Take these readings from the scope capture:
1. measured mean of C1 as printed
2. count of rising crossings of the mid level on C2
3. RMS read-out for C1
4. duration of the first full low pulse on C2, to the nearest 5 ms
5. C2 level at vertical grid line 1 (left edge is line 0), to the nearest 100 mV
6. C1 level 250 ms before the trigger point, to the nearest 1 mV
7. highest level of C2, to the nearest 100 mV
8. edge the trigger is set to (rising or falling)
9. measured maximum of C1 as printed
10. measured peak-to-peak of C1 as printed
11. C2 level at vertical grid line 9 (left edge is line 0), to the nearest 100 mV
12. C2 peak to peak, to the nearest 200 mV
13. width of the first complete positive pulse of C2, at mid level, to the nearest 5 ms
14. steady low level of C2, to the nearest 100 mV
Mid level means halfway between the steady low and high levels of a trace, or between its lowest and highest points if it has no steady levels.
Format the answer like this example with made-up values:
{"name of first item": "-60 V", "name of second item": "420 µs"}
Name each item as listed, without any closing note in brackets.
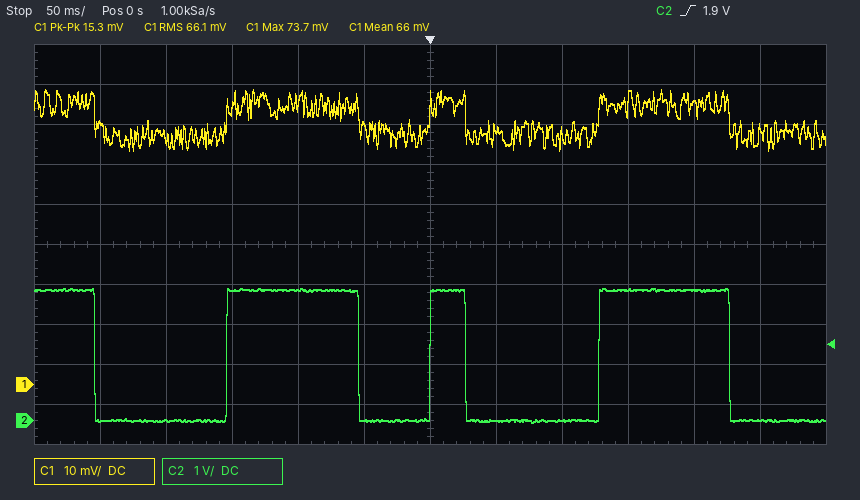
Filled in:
{"measured mean of C1 as printed": "66 mV", "count of rising crossings of the mid level on C2": "3", "RMS read-out for C1": "66.1 mV", "duration of the first full low pulse on C2, to the nearest 5 ms": "100 ms", "C2 level at vertical grid line 1 (left edge is line 0), to the nearest 100 mV": "0.0 V", "C1 level 250 ms before the trigger point, to the nearest 1 mV": "65 mV", "highest level of C2, to the nearest 100 mV": "3.3 V", "edge the trigger is set to": "rising", "measured maximum of C1 as printed": "73.7 mV", "measured peak-to-peak of C1 as printed": "15.3 mV", "C2 level at vertical grid line 9 (left edge is line 0), to the nearest 100 mV": "3.3 V", "C2 peak to peak, to the nearest 200 mV": "3.4 V", "width of the first complete positive pulse of C2, at mid level, to the nearest 5 ms": "100 ms", "steady low level of C2, to the nearest 100 mV": "0.0 V"}
